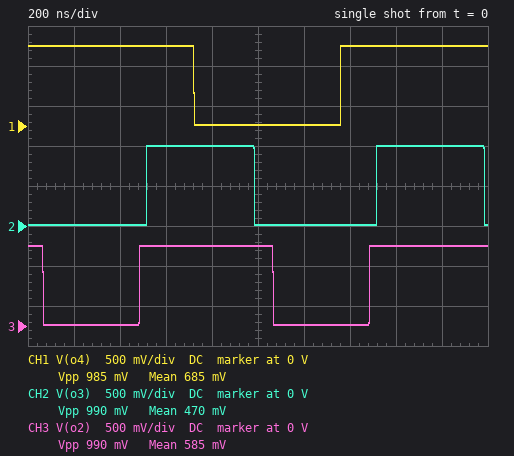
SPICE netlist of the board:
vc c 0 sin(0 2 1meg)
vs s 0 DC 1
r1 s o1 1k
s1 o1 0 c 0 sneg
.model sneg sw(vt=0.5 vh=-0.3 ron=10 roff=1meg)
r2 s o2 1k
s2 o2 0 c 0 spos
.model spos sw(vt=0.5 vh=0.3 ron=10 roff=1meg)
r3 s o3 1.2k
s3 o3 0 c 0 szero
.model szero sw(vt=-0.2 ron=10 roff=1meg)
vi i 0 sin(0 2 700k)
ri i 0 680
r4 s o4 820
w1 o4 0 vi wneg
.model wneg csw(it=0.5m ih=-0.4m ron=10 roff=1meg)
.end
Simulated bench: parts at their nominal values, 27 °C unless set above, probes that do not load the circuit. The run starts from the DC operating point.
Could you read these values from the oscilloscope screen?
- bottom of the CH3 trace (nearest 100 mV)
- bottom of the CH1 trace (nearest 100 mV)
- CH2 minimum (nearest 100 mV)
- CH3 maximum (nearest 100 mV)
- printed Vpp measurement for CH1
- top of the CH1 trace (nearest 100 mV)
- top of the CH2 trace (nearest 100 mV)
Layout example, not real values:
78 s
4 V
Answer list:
0 V
0 V
0 V
1.0 V
985 mV
1.0 V
1.0 V
